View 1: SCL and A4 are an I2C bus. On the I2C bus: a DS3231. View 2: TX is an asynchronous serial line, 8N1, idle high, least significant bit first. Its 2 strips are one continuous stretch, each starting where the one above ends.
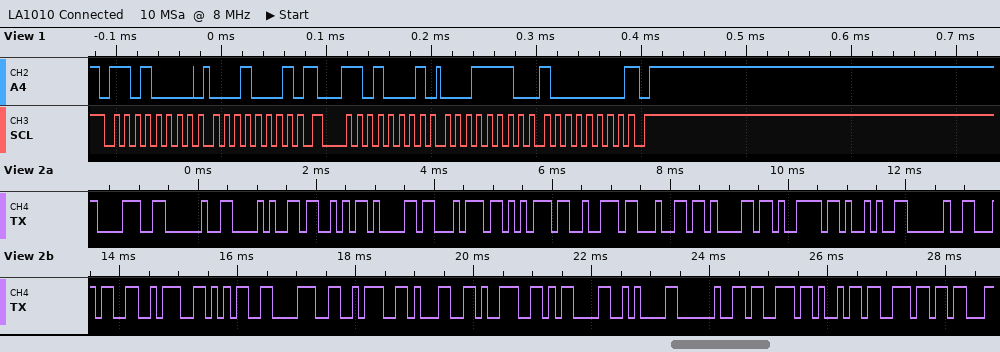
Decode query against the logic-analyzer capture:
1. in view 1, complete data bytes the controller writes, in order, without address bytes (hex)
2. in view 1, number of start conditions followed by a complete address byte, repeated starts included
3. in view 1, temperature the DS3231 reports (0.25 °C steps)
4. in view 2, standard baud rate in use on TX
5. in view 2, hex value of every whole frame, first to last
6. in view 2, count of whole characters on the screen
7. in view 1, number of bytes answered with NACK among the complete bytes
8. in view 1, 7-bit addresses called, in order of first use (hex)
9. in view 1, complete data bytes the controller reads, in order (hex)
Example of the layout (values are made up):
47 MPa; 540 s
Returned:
11; 2; 30.50 °C; 9600 baud; 38 20 28 53 61 74 75 72 64 61 79 29 20 34 3A 35 38 3A 31 39 0D 0A 20 73 69 6E; 26; 1; 0x68; 1E 80
